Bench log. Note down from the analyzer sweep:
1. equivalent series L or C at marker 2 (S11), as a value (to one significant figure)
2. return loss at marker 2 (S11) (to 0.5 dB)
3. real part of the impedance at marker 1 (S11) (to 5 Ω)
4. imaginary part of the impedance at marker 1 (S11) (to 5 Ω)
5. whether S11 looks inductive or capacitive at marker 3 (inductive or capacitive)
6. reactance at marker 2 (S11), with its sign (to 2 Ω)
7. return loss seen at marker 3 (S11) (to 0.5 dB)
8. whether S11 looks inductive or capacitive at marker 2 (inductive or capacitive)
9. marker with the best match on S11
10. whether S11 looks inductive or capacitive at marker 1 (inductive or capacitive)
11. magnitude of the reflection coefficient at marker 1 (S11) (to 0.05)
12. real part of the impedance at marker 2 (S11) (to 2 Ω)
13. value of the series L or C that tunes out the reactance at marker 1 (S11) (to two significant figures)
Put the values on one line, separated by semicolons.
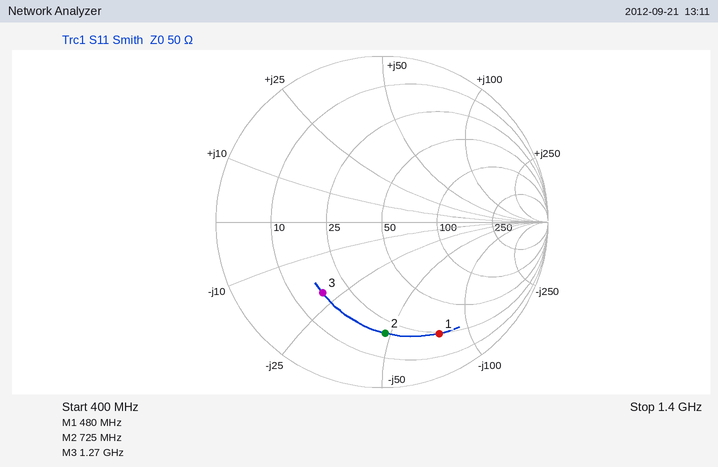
5 pF; 3.5 dB; 25 Ω; -75 Ω; capacitive; -48 Ω; 5.0 dB; capacitive; marker 3; capacitive; 0.75; 20 Ω; 25 nH
